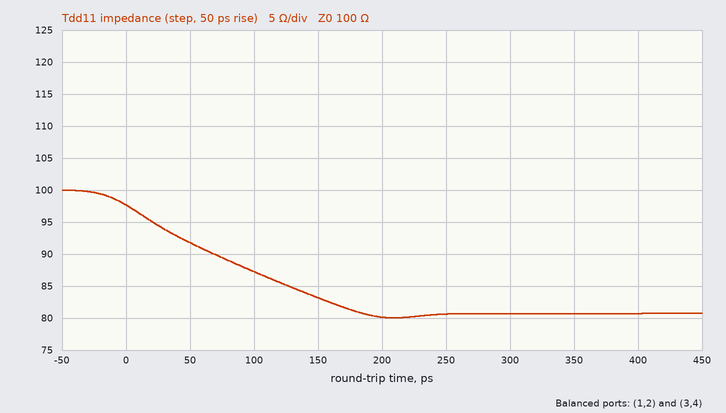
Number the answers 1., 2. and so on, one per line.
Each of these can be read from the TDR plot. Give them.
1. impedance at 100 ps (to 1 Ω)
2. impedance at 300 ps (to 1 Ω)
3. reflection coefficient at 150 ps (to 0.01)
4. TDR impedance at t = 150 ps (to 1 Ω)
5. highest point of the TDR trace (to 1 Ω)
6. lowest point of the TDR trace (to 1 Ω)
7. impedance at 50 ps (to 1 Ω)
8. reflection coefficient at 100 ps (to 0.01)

1. 87 Ω
2. 81 Ω
3. -0.09
4. 83 Ω
5. 100 Ω
6. 80 Ω
7. 92 Ω
8. -0.07
